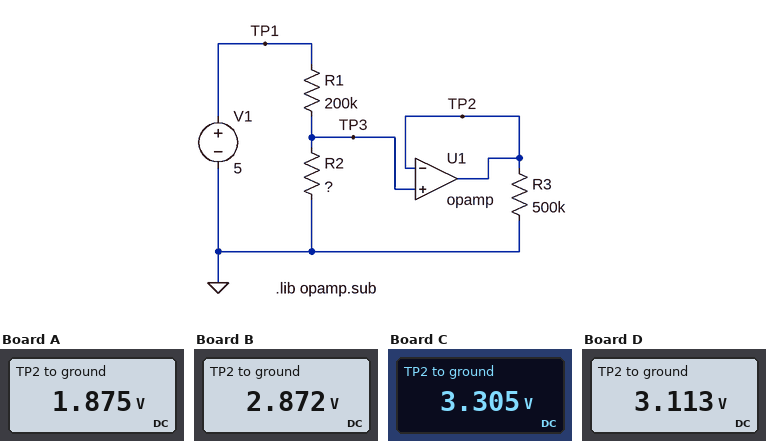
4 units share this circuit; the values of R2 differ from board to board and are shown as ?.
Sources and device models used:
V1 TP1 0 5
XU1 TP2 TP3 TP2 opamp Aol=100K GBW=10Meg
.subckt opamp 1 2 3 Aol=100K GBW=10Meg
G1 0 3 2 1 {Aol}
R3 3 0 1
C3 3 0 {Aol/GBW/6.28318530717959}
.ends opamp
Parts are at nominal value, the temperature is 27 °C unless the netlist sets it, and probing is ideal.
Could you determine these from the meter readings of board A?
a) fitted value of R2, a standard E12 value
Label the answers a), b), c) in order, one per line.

a) 120 kΩ
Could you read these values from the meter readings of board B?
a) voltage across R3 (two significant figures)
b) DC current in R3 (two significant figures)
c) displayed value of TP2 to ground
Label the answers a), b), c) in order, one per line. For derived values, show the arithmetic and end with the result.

a) 2.872 V = 2.9 V
b) (2.872 V) / 500 kΩ = 5.7 µA
c) 2.872 V
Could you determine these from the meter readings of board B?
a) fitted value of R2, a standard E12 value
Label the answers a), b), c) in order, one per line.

a) 270 kΩ
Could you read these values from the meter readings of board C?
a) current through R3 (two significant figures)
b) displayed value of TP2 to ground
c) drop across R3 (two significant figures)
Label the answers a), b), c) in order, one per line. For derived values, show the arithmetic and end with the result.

a) (3.305 V) / 500 kΩ = 6.6 µA
b) 3.305 V
c) 3.305 V = 3.3 V
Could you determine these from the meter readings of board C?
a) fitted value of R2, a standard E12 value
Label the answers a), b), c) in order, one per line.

a) 390 kΩ
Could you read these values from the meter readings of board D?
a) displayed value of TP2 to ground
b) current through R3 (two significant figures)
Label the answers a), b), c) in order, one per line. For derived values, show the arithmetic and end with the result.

a) 3.113 V
b) (3.113 V) / 500 kΩ = 6.2 µA
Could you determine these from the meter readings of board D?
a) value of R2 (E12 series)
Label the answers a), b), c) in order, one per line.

a) 330 kΩ
